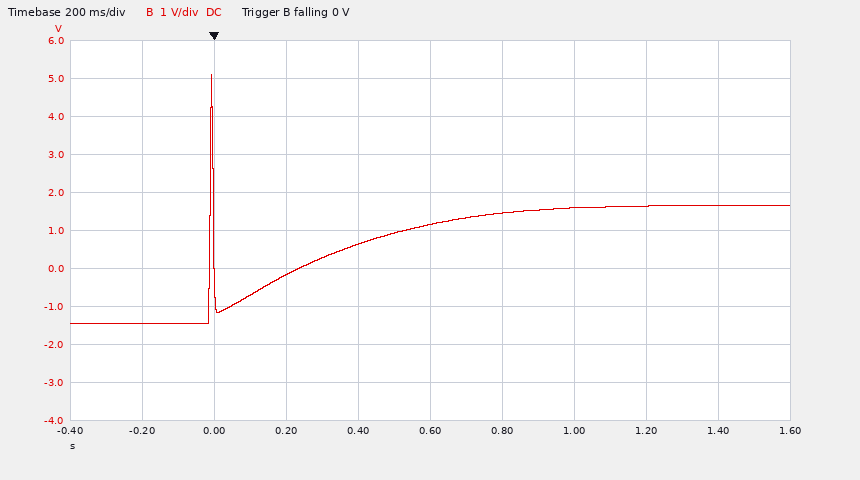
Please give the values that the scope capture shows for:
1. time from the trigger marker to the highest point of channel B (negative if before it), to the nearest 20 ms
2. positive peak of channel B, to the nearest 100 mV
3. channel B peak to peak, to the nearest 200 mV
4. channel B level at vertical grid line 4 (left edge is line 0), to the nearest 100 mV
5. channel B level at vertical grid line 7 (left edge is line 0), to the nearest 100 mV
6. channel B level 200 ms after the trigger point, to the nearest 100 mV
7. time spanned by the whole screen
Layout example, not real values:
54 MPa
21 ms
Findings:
0 ms
5.1 V
6.6 V
600 mV
1.6 V
-200 mV
2 s
